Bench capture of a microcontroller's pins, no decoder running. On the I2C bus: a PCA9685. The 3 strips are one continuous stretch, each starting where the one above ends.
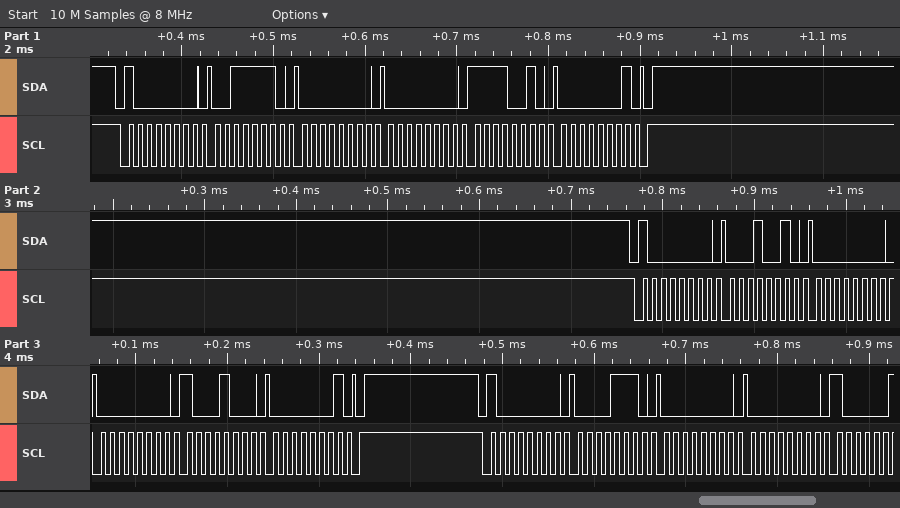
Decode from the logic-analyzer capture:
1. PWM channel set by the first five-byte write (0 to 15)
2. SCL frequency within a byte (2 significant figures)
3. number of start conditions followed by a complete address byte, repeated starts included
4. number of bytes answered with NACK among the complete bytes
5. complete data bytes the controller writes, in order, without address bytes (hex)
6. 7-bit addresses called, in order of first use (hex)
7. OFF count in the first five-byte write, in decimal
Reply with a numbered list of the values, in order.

1. 14
2. 100 kHz
3. 3
4. 0
5. 3E 00 00 F2 01 12 00 00 88 01 0E 00 00
6. 0x40
7. 498
